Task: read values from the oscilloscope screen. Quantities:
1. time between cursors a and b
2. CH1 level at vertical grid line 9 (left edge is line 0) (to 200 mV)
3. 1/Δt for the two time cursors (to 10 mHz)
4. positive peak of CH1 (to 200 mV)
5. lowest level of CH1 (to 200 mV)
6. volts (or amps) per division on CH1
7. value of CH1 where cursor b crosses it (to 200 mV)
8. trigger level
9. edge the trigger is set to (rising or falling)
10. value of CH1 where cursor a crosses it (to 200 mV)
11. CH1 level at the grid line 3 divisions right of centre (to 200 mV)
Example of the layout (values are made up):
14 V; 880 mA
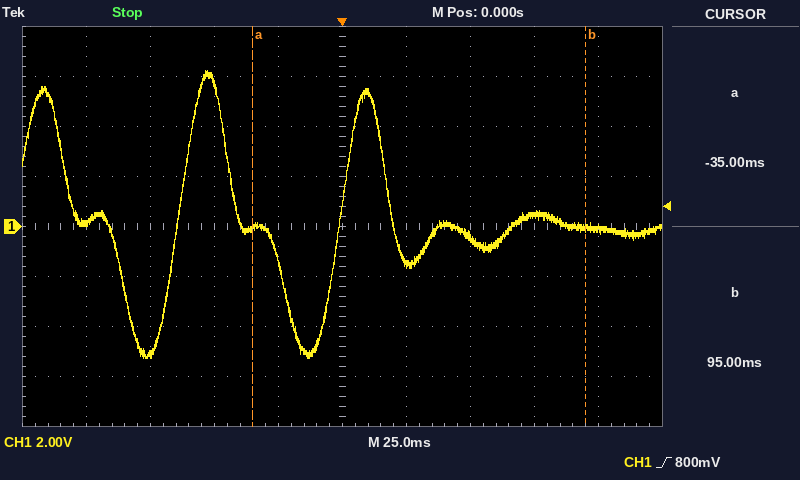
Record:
130.0 ms; -200 mV; 7.69 Hz; 6.2 V; -5.2 V; 2 V; 0.0 V; 800 mV; rising; 0.0 V; 400 mV
